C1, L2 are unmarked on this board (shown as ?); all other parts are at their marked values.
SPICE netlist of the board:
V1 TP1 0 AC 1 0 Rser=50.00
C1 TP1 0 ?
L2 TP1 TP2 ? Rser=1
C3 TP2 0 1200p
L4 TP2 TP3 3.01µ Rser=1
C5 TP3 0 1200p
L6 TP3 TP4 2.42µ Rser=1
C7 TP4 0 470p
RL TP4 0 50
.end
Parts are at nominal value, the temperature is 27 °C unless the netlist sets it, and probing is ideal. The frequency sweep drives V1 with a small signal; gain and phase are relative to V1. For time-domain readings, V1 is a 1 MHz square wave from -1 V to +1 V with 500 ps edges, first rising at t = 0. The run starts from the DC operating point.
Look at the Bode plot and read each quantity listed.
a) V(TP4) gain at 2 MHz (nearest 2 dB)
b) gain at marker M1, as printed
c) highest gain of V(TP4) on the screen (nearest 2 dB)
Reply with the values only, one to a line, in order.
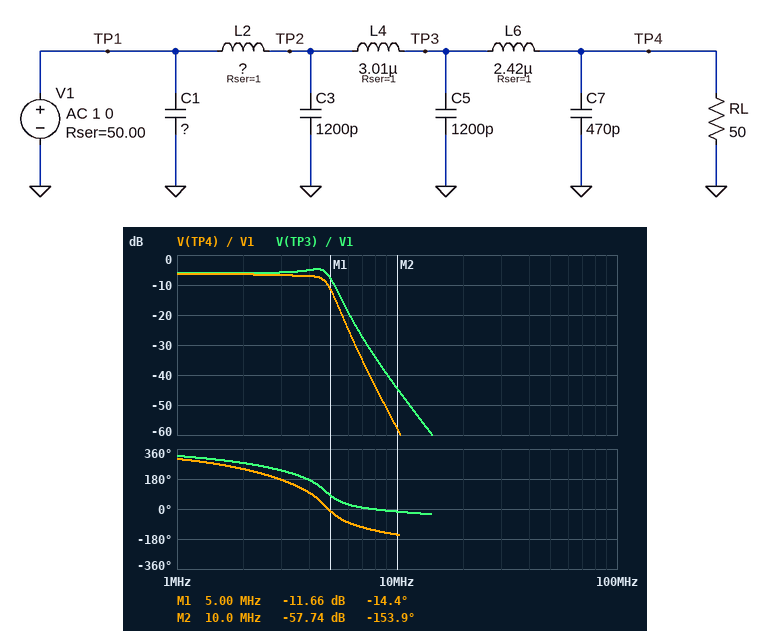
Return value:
-6 dB
-11.66 dB
-6 dB
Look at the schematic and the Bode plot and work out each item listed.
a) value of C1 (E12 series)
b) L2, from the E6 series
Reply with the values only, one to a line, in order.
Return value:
180 pF
3.3 µH
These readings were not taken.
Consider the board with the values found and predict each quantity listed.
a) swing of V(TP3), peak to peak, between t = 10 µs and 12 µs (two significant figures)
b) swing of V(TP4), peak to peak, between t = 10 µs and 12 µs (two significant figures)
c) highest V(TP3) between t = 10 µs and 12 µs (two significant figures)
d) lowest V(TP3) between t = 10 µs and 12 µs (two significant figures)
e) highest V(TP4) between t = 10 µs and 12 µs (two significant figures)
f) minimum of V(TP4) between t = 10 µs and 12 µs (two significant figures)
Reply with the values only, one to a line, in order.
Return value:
1.4 V
1.3 V
680 mV
-680 mV
630 mV
-630 mV
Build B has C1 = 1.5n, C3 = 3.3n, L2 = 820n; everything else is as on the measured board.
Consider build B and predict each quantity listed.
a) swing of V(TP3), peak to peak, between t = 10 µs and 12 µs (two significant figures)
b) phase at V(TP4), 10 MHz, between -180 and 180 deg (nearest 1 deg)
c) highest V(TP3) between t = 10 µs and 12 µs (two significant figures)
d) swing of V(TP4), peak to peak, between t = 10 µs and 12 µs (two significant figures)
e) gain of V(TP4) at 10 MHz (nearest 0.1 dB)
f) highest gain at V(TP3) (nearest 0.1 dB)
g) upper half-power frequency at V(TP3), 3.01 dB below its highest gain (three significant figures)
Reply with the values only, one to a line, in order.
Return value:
990 mV
150 deg
490 mV
950 mV
-65.8 dB
-6.1 dB
1.85 MHz
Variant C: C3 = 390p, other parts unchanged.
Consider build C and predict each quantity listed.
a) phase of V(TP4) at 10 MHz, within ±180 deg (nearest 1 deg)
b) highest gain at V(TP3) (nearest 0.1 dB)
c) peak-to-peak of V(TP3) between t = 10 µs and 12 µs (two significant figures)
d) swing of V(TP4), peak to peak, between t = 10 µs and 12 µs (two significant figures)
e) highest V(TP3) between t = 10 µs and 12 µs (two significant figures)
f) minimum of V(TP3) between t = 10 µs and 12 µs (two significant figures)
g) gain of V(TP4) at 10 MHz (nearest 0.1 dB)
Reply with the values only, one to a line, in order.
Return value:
-150 deg
-4.5 dB
1.2 V
1.0 V
610 mV
-610 mV
-44.3 dB
